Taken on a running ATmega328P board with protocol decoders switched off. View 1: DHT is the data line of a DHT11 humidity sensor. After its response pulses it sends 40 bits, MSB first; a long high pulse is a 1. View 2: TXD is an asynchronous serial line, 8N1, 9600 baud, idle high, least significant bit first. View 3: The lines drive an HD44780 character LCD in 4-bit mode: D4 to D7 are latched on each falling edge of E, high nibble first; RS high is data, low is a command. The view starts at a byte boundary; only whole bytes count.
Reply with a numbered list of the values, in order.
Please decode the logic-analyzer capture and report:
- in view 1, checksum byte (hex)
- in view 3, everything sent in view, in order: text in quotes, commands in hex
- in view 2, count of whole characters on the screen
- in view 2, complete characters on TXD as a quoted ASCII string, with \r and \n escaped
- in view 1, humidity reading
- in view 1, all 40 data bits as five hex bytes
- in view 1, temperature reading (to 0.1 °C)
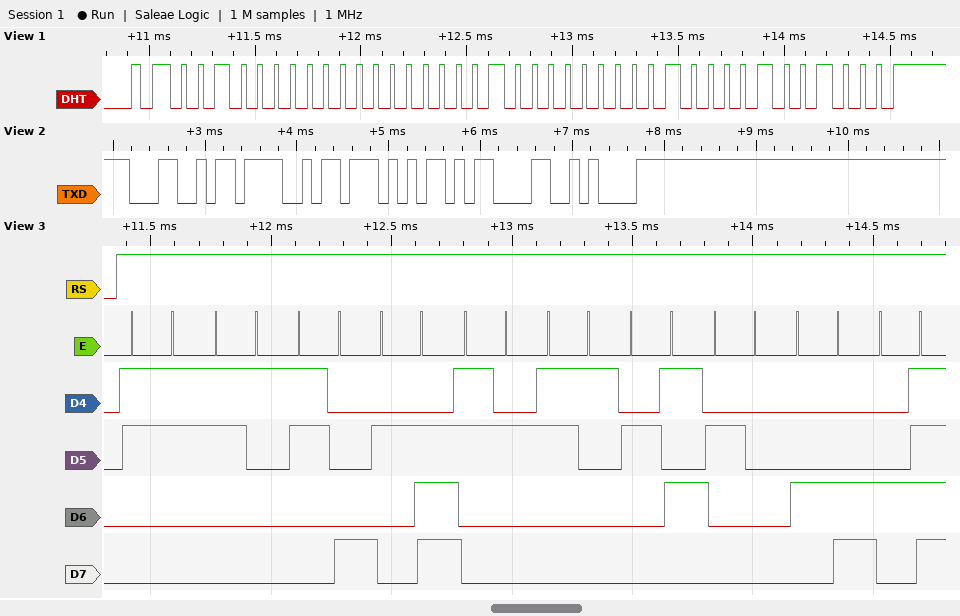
1. 0x48
2. "318.21% LO"
3. 5
4. "LOW\r\n"
5. 32 %
6. 20 00 20 08 48
7. 32.8 °C
